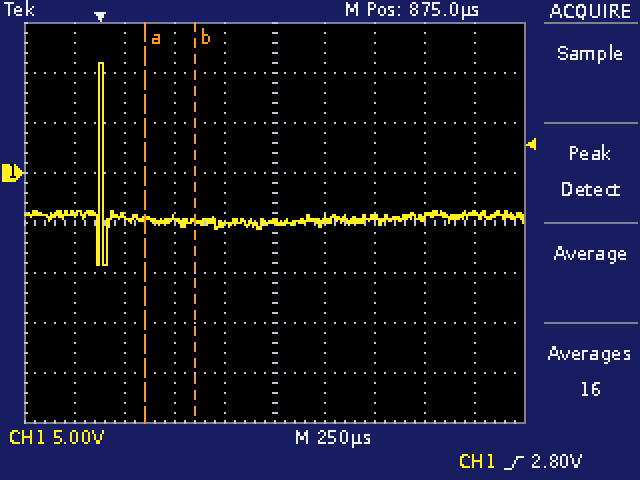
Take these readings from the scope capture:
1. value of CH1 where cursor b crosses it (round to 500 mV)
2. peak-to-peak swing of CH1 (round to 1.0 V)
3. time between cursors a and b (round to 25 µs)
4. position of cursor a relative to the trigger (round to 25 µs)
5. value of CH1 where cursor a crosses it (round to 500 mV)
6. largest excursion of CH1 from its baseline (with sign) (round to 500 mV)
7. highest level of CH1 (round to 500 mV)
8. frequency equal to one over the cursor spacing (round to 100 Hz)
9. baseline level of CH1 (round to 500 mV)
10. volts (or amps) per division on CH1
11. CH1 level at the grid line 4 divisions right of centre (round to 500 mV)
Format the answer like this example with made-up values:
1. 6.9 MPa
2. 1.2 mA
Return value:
1. -5.0 V
2. 20.0 V
3. 250 µs
4. +225 µs
5. -4.5 V
6. +15.5 V
7. 11.0 V
8. 4.0 kHz
9. -4.5 V
10. 5 V
11. -4.0 V
